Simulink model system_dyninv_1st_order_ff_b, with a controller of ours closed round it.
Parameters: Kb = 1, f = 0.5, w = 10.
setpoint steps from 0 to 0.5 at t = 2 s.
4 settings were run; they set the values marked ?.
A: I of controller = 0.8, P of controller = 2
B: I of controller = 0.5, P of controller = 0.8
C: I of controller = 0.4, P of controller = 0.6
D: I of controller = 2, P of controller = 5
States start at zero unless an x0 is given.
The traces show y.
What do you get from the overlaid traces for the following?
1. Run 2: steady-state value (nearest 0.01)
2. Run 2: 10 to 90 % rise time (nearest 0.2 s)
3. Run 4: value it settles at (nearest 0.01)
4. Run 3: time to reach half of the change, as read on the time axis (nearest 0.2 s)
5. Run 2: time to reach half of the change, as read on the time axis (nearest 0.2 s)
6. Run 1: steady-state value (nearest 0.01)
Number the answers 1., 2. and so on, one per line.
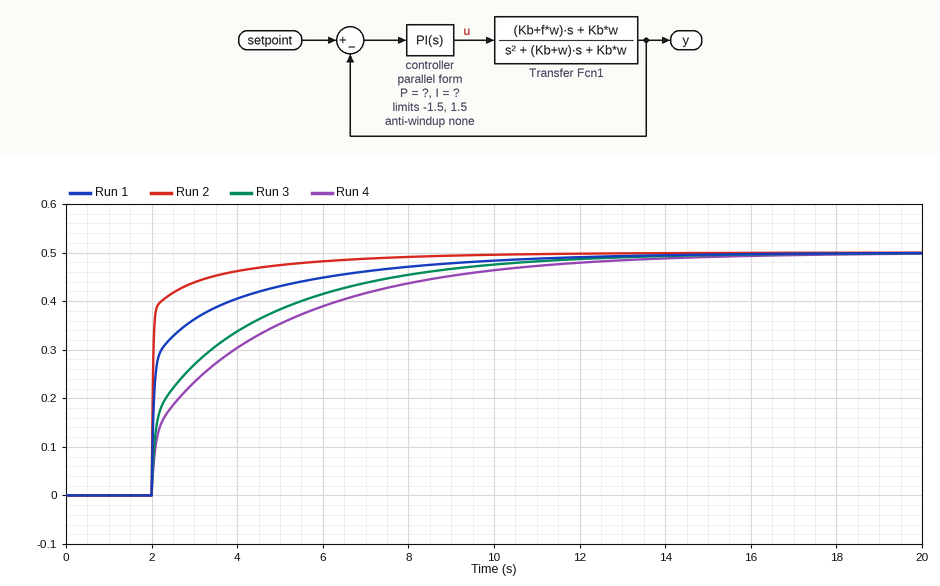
1. 0.50
2. 1.4 s
3. 0.50
4. 2.8 s
5. 2.0 s
6. 0.50
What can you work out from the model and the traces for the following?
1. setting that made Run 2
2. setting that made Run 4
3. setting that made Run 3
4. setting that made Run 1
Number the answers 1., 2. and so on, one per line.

1. D
2. C
3. B
4. A
